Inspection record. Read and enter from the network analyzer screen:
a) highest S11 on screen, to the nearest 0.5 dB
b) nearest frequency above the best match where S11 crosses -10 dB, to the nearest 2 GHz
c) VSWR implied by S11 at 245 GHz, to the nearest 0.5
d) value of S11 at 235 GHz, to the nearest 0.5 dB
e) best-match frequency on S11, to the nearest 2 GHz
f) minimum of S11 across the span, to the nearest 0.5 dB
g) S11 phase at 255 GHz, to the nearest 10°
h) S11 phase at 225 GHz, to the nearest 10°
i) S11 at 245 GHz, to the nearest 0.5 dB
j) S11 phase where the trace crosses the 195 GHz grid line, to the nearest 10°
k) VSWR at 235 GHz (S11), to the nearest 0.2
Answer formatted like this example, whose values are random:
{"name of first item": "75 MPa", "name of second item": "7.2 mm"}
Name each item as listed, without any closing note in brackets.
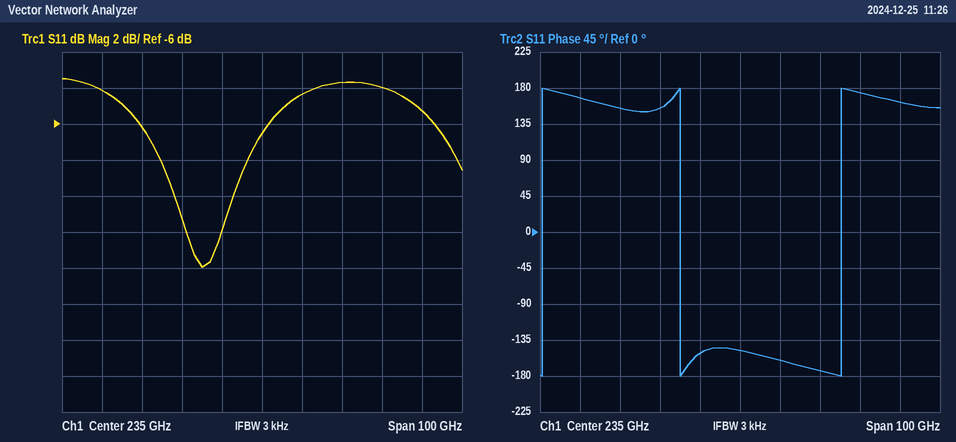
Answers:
{"highest S11 on screen, to the nearest 0.5 dB": "-3.5 dB", "nearest frequency above the best match where S11 crosses -10 dB, to the nearest 2 GHz": "228 GHz", "VSWR implied by S11 at 245 GHz, to the nearest 0.5": "4.0", "value of S11 at 235 GHz, to the nearest 0.5 dB": "-6.5 dB", "best-match frequency on S11, to the nearest 2 GHz": "220 GHz", "minimum of S11 across the span, to the nearest 0.5 dB": "-14.0 dB", "S11 phase at 255 GHz, to the nearest 10°": "-170°", "S11 phase at 225 GHz, to the nearest 10°": "-150°", "S11 at 245 GHz, to the nearest 0.5 dB": "-4.5 dB", "S11 phase where the trace crosses the 195 GHz grid line, to the nearest 10°": "170°", "VSWR at 235 GHz (S11), to the nearest 0.2": "2.8"}
